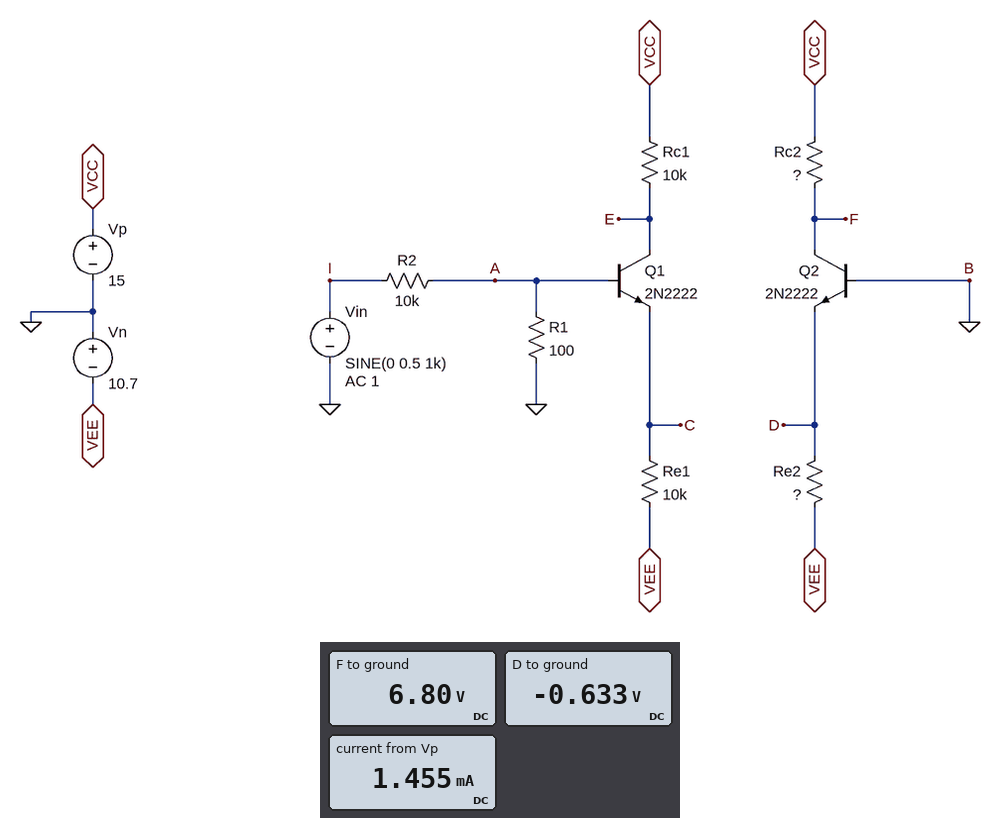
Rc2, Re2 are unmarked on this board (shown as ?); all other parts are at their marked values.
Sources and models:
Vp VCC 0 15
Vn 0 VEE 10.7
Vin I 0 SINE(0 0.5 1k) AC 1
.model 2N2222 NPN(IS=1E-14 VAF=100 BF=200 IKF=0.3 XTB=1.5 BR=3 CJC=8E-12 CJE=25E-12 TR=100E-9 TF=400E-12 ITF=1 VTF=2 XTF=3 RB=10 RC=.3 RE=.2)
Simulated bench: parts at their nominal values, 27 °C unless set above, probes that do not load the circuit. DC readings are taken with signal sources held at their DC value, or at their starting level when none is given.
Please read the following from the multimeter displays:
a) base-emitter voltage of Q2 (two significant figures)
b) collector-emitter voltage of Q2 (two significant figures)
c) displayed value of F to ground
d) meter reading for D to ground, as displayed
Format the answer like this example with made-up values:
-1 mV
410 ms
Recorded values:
630 mV
7.4 V
6.80 V
-0.633 V
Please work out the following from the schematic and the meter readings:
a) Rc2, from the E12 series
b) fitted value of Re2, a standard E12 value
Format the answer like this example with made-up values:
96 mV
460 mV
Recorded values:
18 kΩ
22 kΩ
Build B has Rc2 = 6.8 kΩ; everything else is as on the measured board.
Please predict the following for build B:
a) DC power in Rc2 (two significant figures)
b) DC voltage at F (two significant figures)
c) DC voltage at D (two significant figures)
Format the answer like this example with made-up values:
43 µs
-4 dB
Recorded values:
1.4 mW
12 V
-630 mV
